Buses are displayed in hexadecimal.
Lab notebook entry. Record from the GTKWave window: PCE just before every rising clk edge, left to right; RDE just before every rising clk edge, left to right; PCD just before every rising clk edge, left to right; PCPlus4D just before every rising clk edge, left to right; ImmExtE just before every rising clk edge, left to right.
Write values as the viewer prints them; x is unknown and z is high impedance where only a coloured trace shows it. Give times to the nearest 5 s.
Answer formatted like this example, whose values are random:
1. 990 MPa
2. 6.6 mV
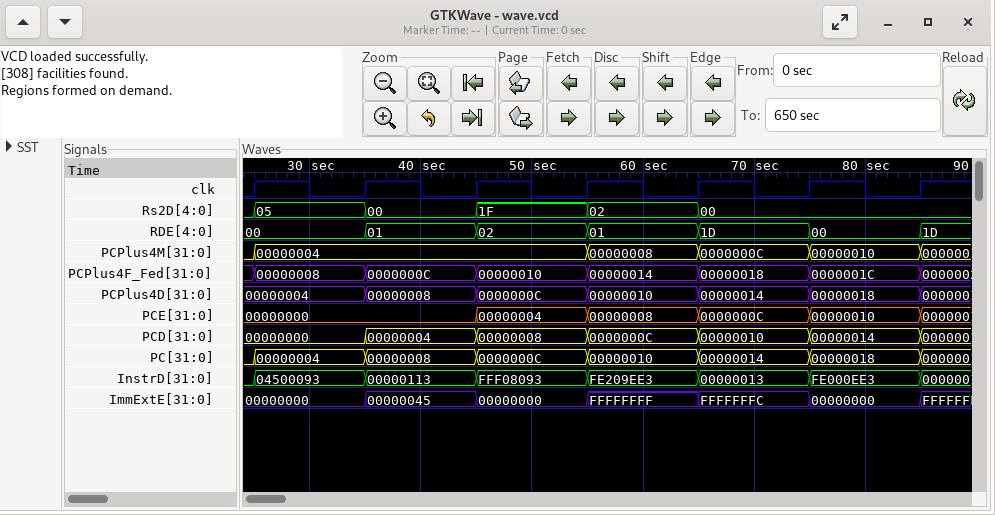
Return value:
1. 00000000, 00000000, 00000000, 00000004, 00000008, 0000000C, 00000010
2. 00, 00, 01, 02, 01, 1D, 00
3. 00000000, 00000000, 00000004, 00000008, 0000000C, 00000010, 00000014
4. 00000004, 00000004, 00000008, 0000000C, 00000010, 00000014, 00000018
5. 00000000, 00000000, 00000045, 00000000, FFFFFFFF, FFFFFFFC, 00000000
